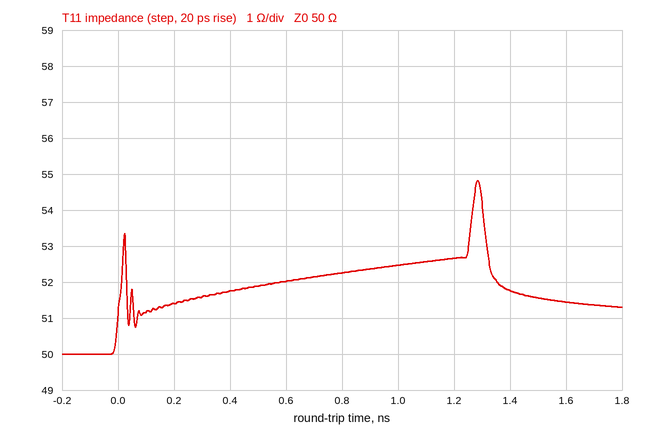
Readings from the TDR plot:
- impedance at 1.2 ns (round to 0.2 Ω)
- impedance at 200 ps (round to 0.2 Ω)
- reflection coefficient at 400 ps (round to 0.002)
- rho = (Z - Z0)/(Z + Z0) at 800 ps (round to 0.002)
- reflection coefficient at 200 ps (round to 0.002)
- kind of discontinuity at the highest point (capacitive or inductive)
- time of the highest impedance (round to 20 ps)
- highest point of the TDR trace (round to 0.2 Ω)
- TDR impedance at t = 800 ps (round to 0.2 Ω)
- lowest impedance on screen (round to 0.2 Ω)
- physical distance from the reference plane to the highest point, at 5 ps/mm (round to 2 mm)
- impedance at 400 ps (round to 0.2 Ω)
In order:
52.6 Ω
51.4 Ω
+0.018
+0.022
+0.014
inductive
1.28 ns
54.8 Ω
52.2 Ω
50.0 Ω
128 mm
51.8 Ω
